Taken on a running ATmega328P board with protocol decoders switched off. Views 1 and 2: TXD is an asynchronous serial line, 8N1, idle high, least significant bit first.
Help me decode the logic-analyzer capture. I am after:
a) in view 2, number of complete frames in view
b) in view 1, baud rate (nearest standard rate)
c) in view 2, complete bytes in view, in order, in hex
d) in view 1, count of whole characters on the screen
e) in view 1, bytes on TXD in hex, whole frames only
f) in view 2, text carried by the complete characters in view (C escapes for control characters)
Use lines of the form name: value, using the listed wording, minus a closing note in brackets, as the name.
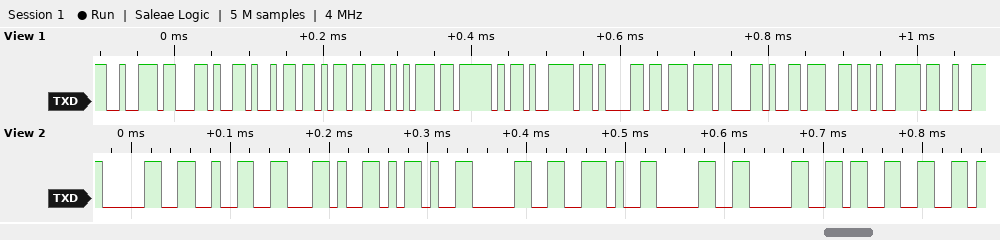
in view 2, number of complete frames in view: 9
in view 1, baud rate: 115200 baud
in view 2, complete bytes in view, in order, in hex: 30 32 2C 2D 30 2E 30 30 33
in view 1, count of whole characters on the screen: 12
in view 1, bytes on TXD in hex, whole frames only: 72 2C 69 6D 75 5F 79 61 77 2C 67 79
in view 2, text carried by the complete characters in view: "02,-0.003"
